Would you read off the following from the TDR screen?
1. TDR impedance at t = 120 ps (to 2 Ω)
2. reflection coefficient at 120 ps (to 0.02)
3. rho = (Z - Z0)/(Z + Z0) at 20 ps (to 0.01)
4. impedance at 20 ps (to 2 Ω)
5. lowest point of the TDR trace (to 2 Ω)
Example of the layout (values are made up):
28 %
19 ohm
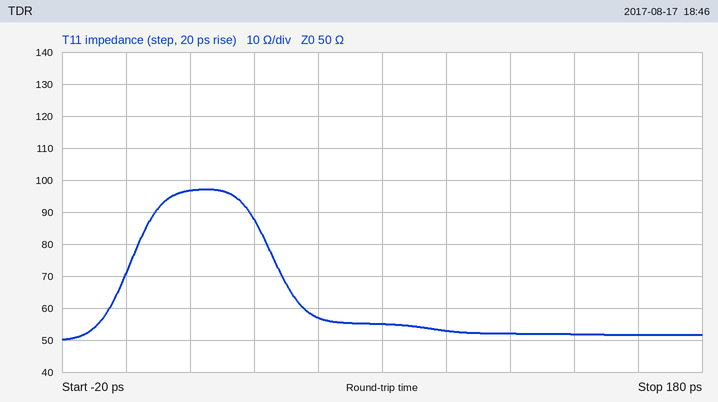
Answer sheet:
52 Ω
+0.02
+0.32
96 Ω
50 Ω
